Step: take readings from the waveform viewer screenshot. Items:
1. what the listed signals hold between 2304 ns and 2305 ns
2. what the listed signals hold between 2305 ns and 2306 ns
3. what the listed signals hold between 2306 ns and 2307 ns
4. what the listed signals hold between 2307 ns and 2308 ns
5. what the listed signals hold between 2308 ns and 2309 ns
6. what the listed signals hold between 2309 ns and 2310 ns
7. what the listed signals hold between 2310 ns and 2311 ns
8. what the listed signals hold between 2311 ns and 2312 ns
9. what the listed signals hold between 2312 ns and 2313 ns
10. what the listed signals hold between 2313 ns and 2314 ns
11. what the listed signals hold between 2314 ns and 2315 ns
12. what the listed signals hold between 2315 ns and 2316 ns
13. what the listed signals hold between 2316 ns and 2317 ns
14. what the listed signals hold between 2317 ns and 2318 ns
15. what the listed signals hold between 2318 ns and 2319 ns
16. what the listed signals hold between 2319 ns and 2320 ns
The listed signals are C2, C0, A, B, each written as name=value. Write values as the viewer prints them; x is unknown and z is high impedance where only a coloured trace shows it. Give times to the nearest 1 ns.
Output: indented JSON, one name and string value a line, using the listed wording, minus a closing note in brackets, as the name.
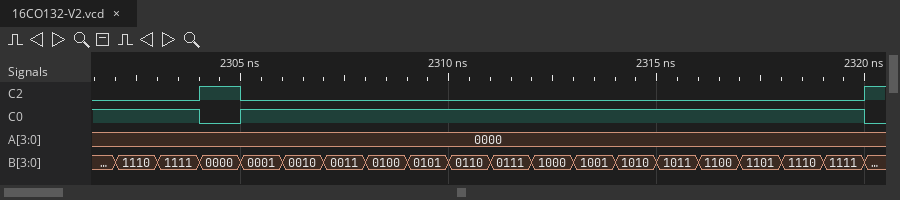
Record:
{
  "what the listed signals hold between 2304 ns and 2305 ns": "C2=1, C0=0, A=0000, B=0000",
  "what the listed signals hold between 2305 ns and 2306 ns": "C2=0, C0=1, A=0000, B=0001",
  "what the listed signals hold between 2306 ns and 2307 ns": "C2=0, C0=1, A=0000, B=0010",
  "what the listed signals hold between 2307 ns and 2308 ns": "C2=0, C0=1, A=0000, B=0011",
  "what the listed signals hold between 2308 ns and 2309 ns": "C2=0, C0=1, A=0000, B=0100",
  "what the listed signals hold between 2309 ns and 2310 ns": "C2=0, C0=1, A=0000, B=0101",
  "what the listed signals hold between 2310 ns and 2311 ns": "C2=0, C0=1, A=0000, B=0110",
  "what the listed signals hold between 2311 ns and 2312 ns": "C2=0, C0=1, A=0000, B=0111",
  "what the listed signals hold between 2312 ns and 2313 ns": "C2=0, C0=1, A=0000, B=1000",
  "what the listed signals hold between 2313 ns and 2314 ns": "C2=0, C0=1, A=0000, B=1001",
  "what the listed signals hold between 2314 ns and 2315 ns": "C2=0, C0=1, A=0000, B=1010",
  "what the listed signals hold between 2315 ns and 2316 ns": "C2=0, C0=1, A=0000, B=1011",
  "what the listed signals hold between 2316 ns and 2317 ns": "C2=0, C0=1, A=0000, B=1100",
  "what the listed signals hold between 2317 ns and 2318 ns": "C2=0, C0=1, A=0000, B=1101",
  "what the listed signals hold between 2318 ns and 2319 ns": "C2=0, C0=1, A=0000, B=1110",
  "what the listed signals hold between 2319 ns and 2320 ns": "C2=0, C0=1, A=0000, B=1111"
}
